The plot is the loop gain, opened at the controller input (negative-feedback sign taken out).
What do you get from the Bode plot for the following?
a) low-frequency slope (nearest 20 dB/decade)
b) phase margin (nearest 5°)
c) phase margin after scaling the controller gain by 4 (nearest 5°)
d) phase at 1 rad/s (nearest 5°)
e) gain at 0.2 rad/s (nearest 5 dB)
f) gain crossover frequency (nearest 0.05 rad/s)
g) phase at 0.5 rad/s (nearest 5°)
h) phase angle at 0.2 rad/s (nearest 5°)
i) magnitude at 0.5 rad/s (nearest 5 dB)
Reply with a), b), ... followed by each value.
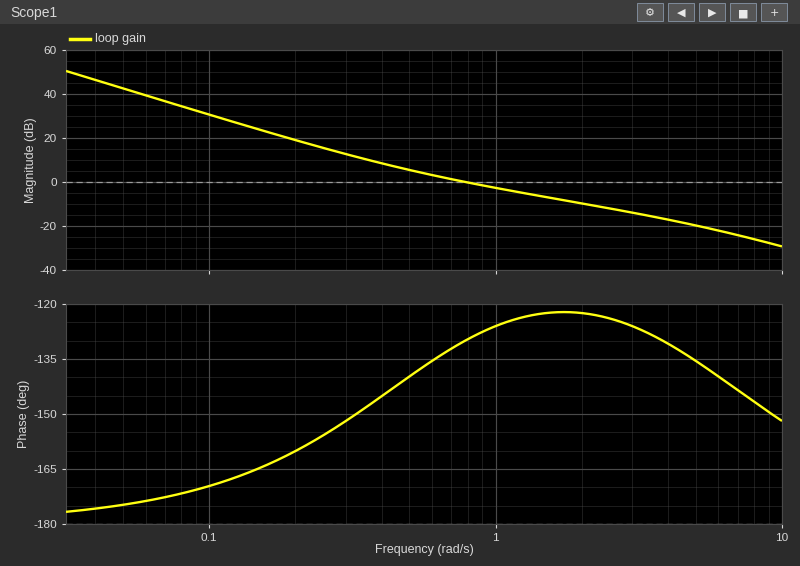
a) -40 dB/decade
b) 50°
c) 55°
d) -125°
e) 20 dB
f) 0.80 rad/s
g) -140°
h) -160°
i) 5 dB
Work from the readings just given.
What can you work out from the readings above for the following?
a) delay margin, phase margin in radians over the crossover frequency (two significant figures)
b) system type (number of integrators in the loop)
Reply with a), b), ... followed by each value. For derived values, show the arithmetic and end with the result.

a) 50 × π / 180 / 0.8 = 1.1 s
b) 2
